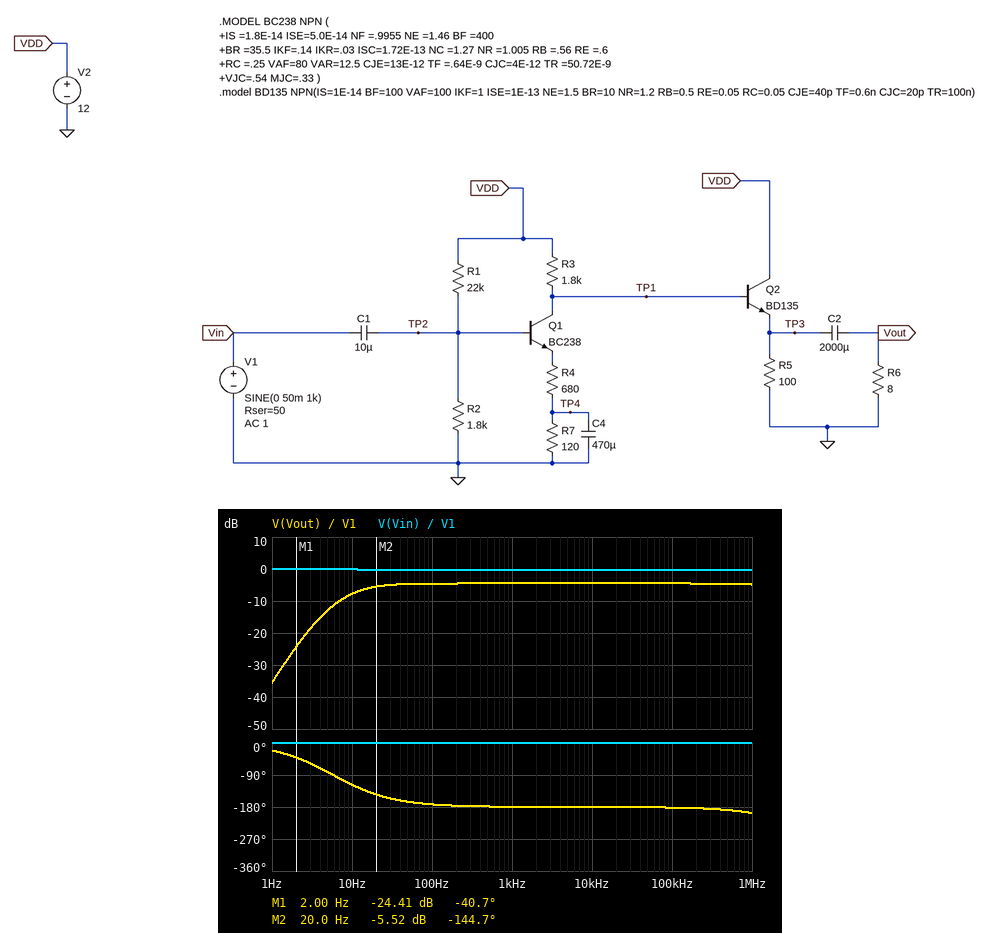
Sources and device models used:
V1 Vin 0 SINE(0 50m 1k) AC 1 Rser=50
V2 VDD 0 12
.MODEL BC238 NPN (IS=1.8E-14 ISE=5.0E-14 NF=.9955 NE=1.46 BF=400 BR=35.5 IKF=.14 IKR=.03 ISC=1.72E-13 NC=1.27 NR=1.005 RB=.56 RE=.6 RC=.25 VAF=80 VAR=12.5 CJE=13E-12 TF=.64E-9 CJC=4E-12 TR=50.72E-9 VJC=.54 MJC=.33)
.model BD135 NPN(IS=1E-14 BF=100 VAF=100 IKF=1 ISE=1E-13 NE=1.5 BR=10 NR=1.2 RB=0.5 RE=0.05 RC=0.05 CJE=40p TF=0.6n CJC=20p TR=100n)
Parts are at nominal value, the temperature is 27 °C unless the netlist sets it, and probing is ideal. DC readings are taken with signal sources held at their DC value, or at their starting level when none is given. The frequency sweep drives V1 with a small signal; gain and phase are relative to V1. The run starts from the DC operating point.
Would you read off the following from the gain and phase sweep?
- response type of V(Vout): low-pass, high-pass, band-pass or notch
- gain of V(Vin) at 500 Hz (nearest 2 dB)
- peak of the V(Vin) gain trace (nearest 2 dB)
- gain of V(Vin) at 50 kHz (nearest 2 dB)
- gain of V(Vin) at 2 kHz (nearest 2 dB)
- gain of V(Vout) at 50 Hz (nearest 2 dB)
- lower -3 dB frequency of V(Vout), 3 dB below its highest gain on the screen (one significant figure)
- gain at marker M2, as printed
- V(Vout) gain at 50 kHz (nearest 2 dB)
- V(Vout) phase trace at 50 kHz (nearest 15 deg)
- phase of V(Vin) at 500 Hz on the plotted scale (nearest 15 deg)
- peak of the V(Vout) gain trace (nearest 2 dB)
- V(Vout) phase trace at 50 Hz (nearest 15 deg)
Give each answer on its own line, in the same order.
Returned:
high-pass
0 dB
0 dB
0 dB
0 dB
-4 dB
10 Hz
-5.52 dB
-4 dB
-180 deg
0 deg
-4 dB
-165 deg
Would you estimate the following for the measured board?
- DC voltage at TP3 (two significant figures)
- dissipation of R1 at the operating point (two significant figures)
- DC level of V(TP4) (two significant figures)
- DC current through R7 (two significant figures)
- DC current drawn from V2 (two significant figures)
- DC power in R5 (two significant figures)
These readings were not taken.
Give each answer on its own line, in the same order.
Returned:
8.8 V
5.6 mW
44 mV
370 µA
89 mA
780 mW
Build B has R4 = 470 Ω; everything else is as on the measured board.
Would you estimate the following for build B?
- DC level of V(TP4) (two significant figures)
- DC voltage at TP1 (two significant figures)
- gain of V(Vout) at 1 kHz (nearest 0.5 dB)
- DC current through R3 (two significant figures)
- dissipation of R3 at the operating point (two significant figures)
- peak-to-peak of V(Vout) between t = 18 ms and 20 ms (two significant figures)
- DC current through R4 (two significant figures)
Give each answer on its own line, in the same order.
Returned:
58 mV
9.4 V
-1.5 dB
1.4 mA
3.7 mW
85 mV
490 µA
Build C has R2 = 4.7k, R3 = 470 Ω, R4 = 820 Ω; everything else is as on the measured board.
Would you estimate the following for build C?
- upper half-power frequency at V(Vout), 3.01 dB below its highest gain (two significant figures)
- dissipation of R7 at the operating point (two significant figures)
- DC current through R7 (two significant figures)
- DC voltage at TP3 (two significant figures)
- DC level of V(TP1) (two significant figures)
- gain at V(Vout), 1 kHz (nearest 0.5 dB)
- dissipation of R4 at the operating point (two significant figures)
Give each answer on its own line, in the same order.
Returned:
6.1 MHz
280 µW
1.5 mA
10 V
11 V
-10.5 dB
1.9 mW
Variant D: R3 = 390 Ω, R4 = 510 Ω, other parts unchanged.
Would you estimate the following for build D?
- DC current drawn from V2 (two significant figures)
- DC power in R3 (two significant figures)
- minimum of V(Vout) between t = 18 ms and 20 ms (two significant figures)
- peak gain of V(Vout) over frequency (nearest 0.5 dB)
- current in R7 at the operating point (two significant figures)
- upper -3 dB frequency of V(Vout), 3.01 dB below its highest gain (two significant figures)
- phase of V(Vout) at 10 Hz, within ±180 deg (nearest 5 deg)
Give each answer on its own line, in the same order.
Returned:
110 mA
1.1 mW
-20 mV
-8.0 dB
460 µA
6.7 MHz
-100 deg
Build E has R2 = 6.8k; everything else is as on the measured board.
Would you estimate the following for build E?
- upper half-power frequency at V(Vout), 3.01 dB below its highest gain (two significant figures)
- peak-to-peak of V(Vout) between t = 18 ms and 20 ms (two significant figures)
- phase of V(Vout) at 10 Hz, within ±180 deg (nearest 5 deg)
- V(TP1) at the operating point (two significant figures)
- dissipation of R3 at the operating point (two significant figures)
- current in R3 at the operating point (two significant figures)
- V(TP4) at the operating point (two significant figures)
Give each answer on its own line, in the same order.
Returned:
3.3 MHz
70 mV
-140 deg
6.2 V
19 mW
3.2 mA
320 mV
